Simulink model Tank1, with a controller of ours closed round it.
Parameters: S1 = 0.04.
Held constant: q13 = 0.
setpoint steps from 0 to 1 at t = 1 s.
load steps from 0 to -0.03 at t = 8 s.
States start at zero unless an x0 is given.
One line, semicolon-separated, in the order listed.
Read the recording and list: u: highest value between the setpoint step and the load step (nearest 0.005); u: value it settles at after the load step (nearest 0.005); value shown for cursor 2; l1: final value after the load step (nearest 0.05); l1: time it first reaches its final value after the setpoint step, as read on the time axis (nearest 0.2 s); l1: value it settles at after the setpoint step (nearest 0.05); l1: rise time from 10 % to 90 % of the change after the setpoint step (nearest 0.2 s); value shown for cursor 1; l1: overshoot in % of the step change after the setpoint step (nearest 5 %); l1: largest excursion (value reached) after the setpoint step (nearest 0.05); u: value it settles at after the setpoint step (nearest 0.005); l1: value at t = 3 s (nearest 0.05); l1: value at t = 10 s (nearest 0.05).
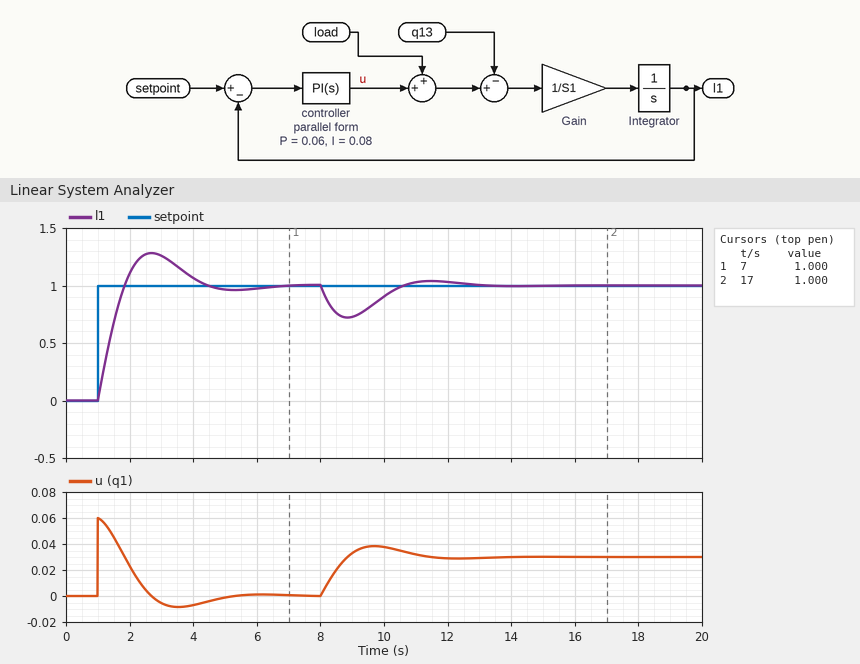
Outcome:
0.060; 0.030; 1.000; 1.00; 1.8 s; 1.00; 0.6 s; 1.000; 30 %; 1.30; 0.000; 1.25; 0.90
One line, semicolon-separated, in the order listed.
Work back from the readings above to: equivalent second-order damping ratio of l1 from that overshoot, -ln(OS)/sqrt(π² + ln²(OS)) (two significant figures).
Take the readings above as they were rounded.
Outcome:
0.36
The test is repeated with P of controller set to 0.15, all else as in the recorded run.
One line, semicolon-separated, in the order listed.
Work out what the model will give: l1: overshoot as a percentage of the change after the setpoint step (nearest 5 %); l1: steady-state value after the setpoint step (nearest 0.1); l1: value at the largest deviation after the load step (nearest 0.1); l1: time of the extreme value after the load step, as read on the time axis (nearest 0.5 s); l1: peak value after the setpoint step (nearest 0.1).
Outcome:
10 %; 1.0; 0.8; 8.5 s; 1.1
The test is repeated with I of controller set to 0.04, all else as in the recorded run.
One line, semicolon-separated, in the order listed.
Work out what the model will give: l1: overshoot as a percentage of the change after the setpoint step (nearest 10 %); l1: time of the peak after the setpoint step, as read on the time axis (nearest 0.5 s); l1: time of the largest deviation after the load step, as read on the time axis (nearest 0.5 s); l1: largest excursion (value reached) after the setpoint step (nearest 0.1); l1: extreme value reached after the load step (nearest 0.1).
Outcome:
20 %; 3.0 s; 9.0 s; 1.2; 0.7
